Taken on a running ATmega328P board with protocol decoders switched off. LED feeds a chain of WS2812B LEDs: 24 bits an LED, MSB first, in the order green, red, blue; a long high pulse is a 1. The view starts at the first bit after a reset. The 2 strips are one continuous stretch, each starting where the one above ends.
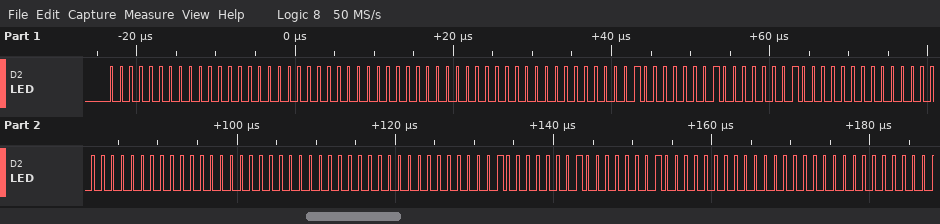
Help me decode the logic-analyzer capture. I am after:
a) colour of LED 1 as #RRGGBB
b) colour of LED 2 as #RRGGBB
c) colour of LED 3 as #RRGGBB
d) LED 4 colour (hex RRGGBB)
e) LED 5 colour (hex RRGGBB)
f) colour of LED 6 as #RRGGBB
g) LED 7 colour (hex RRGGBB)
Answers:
#000000
#000000
#040404
#000000
#000000
#040404
#000000
